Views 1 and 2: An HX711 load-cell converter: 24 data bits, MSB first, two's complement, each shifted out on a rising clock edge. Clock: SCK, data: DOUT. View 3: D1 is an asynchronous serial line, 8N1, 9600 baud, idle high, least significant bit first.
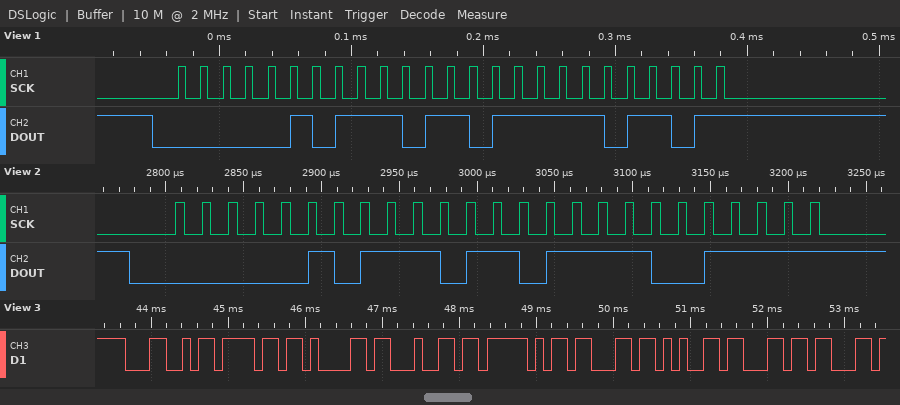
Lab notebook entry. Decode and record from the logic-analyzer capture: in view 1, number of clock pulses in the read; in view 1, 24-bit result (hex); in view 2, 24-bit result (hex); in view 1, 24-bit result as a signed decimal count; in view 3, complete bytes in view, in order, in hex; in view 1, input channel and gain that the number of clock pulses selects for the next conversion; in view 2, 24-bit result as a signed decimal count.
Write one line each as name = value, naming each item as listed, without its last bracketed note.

in view 1, number of clock pulses in the read = 25
in view 1, 24-bit result = 0x05DBED
in view 2, 24-bit result = 0x05DBCF
in view 1, 24-bit result as a signed decimal count = 383981
in view 3, complete bytes in view, in order, in hex = 4C 6F 61 64 5F 63 65 6C
in view 1, input channel and gain that the number of clock pulses selects for the next conversion = channel A, gain 128
in view 2, 24-bit result as a signed decimal count = 383951
